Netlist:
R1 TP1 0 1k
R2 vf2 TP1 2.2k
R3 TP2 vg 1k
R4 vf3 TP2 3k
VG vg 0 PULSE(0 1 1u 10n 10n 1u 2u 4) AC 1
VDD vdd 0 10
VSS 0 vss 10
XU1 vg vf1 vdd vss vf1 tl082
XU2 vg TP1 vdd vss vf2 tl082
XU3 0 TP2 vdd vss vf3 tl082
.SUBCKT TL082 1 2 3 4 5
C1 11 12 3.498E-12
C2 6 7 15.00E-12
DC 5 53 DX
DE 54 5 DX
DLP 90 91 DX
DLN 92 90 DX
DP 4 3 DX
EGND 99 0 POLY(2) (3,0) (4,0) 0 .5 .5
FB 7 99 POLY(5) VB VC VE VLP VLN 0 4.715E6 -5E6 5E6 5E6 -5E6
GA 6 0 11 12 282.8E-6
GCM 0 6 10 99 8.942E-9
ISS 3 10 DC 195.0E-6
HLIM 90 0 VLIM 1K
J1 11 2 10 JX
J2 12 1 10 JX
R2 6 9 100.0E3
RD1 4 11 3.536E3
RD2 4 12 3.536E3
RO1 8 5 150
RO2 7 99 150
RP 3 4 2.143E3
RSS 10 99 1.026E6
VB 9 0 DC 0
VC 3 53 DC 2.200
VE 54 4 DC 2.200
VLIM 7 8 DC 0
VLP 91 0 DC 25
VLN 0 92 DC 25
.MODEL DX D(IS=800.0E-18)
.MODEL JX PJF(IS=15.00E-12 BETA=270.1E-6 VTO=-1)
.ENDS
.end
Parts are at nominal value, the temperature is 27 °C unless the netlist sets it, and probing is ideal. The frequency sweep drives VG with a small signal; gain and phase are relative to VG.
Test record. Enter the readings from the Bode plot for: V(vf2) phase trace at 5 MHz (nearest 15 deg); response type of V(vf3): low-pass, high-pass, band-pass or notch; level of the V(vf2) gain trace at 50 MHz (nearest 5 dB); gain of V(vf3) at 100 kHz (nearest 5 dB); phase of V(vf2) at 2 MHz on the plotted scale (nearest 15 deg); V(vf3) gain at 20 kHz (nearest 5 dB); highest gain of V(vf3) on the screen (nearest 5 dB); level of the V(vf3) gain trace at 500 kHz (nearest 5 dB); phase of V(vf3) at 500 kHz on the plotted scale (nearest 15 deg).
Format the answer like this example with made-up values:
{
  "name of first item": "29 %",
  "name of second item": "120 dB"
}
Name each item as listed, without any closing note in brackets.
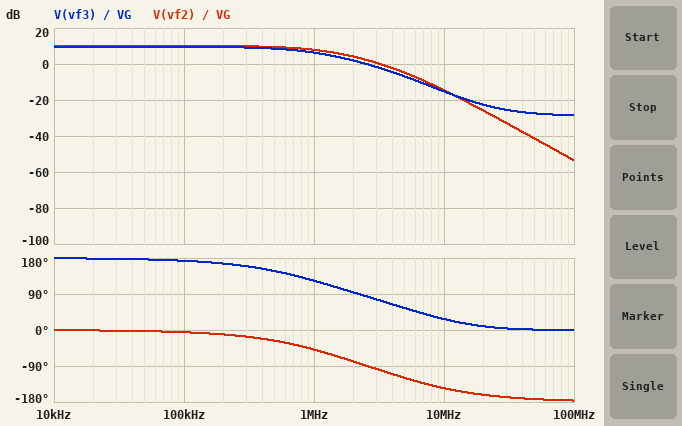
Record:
{
  "V(vf2) phase trace at 5 MHz": "-120 deg",
  "response type of V(vf3): low-pass, high-pass, band-pass or notch": "low-pass",
  "level of the V(vf2) gain trace at 50 MHz": "-40 dB",
  "gain of V(vf3) at 100 kHz": "10 dB",
  "phase of V(vf2) at 2 MHz on the plotted scale": "-75 deg",
  "V(vf3) gain at 20 kHz": "10 dB",
  "highest gain of V(vf3) on the screen": "10 dB",
  "level of the V(vf3) gain trace at 500 kHz": "10 dB",
  "phase of V(vf3) at 500 kHz on the plotted scale": "150 deg"
}
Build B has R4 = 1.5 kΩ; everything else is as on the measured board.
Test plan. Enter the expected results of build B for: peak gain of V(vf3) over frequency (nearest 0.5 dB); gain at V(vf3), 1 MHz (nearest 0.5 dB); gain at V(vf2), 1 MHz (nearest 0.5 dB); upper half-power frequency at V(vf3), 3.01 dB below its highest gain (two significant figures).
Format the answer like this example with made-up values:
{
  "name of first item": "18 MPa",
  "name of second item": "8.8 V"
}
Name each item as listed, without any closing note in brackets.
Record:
{
  "peak gain of V(vf3) over frequency": "3.5 dB",
  "gain at V(vf3), 1 MHz": "2.0 dB",
  "gain at V(vf2), 1 MHz": "8.0 dB",
  "upper half-power frequency at V(vf3), 3.01 dB below its highest gain": "1.6 MHz"
}
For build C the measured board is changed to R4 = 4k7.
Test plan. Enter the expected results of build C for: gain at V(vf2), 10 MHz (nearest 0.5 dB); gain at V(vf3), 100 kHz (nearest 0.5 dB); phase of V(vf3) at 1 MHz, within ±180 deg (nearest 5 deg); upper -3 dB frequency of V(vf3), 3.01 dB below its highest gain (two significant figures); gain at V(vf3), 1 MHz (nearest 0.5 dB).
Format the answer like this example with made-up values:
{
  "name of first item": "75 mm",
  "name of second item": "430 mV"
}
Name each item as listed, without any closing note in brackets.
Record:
{
  "gain at V(vf2), 10 MHz": "-14.5 dB",
  "gain at V(vf3), 100 kHz": "13.5 dB",
  "phase of V(vf3) at 1 MHz, within ±180 deg": "115 deg",
  "upper -3 dB frequency of V(vf3), 3.01 dB below its highest gain": "650 kHz",
  "gain at V(vf3), 1 MHz": "8.0 dB"
}
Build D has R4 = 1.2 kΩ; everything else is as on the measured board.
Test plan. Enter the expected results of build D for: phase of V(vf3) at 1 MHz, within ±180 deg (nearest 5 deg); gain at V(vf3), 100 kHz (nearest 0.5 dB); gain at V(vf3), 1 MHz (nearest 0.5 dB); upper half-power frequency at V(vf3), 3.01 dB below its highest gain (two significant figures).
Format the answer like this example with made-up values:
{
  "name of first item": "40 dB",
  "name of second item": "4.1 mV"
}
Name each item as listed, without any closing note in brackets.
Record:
{
  "phase of V(vf3) at 1 MHz, within ±180 deg": "140 deg",
  "gain at V(vf3), 100 kHz": "1.5 dB",
  "gain at V(vf3), 1 MHz": "0.5 dB",
  "upper half-power frequency at V(vf3), 3.01 dB below its highest gain": "1.9 MHz"
}
